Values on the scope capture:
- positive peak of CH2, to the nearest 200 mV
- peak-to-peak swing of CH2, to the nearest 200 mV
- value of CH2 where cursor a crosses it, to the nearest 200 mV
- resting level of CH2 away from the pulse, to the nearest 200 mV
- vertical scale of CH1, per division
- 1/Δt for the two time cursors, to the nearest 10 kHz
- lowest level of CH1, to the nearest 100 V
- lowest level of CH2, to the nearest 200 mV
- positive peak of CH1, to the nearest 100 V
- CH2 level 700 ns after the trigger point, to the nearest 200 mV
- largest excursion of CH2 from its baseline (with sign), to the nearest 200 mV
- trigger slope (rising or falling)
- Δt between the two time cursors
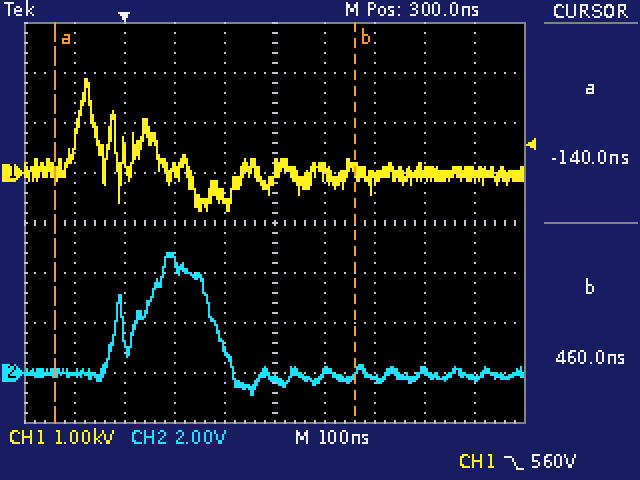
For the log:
4.8 V
5.6 V
0.0 V
0.0 V
1 kV
1.67 MHz
-800 V
-800 mV
1.9 kV
-200 mV
+4.8 V
falling
600 ns
